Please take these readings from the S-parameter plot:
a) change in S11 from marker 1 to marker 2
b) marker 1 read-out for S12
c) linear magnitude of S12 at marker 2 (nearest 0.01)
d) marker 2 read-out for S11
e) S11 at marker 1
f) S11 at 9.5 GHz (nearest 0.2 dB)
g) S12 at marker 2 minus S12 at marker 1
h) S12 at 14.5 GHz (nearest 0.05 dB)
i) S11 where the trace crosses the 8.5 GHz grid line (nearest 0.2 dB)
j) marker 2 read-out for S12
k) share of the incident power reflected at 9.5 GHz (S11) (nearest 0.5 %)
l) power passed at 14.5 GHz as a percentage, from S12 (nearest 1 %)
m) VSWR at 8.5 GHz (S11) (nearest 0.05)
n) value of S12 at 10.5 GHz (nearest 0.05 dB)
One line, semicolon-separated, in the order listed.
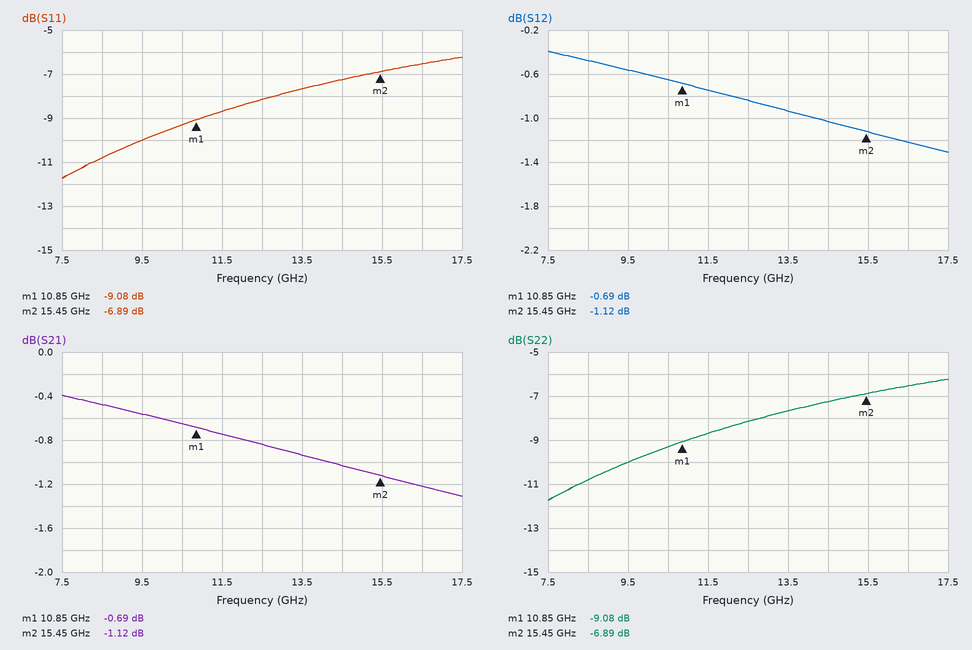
2.19 dB; -0.69 dB; 0.88; -6.89 dB; -9.08 dB; -10.0 dB; -0.43 dB; -1.05 dB; -10.8 dB; -1.12 dB; 10.0 %; 79 %; 1.80; -0.65 dB
